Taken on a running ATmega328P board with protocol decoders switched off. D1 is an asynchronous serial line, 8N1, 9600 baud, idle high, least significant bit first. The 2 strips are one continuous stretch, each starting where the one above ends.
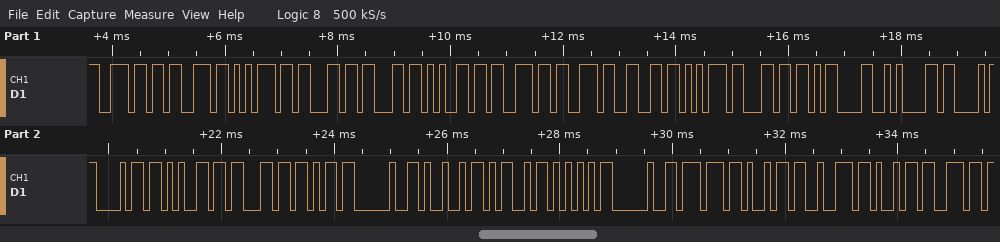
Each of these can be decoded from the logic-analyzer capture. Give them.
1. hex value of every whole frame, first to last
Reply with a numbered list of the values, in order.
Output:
1. 6E 73 75 63 63 65 73 73 66 75 6C 0D 0A 43 68 65 63 6B 20 49 4D 55 20 77 69 72 69 6E
